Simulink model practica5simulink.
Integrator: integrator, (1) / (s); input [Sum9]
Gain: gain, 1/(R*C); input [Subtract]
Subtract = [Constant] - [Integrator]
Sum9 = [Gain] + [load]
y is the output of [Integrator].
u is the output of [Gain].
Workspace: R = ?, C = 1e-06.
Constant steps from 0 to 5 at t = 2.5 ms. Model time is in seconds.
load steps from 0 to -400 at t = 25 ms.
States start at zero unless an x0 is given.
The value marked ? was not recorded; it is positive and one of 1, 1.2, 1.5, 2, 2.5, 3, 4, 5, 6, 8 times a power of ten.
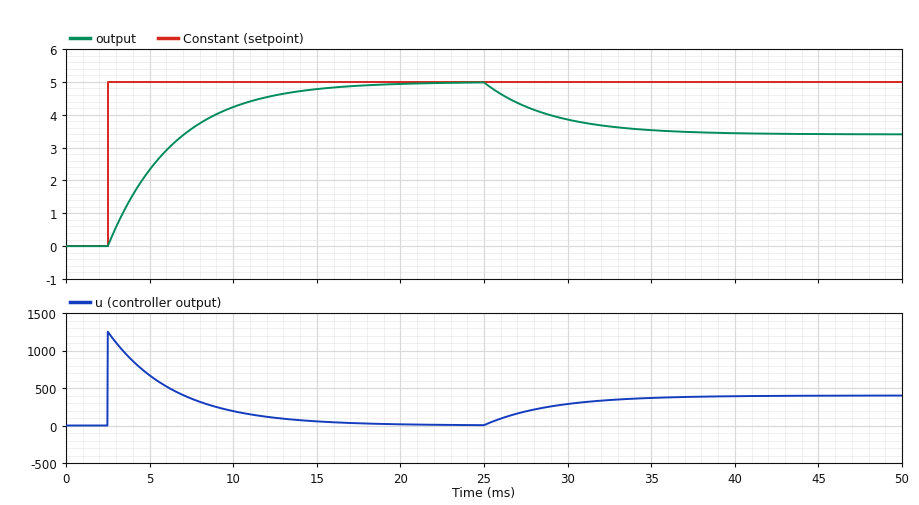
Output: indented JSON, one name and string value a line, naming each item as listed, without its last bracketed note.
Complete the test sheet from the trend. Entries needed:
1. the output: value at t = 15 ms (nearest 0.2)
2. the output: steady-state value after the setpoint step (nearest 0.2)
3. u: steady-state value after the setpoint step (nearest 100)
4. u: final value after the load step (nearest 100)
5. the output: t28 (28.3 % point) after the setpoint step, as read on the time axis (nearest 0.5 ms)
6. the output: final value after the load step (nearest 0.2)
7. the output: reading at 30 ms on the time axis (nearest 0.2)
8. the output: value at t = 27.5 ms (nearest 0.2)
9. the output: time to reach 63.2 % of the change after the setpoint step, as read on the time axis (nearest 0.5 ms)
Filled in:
{
  "the output: value at t = 15 ms": "4.8",
  "the output: steady-state value after the setpoint step": "5.0",
  "u: steady-state value after the setpoint step": "0",
  "u: final value after the load step": "400",
  "the output: t28 (28.3 % point) after the setpoint step, as read on the time axis": "4.0 ms",
  "the output: final value after the load step": "3.4",
  "the output: reading at 30 ms on the time axis": "3.8",
  "the output: value at t = 27.5 ms": "4.2",
  "the output: time to reach 63.2 % of the change after the setpoint step, as read on the time axis": "6.5 ms"
}
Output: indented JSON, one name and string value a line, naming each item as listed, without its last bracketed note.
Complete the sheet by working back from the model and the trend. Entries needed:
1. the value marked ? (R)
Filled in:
{
  "the value marked ?": "4000"
}
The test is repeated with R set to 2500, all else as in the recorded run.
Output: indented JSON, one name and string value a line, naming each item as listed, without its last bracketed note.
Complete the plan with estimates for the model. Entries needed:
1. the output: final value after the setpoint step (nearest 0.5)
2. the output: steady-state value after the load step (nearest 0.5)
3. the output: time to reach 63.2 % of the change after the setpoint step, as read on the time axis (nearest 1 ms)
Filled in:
{
  "the output: final value after the setpoint step": "5.0",
  "the output: steady-state value after the load step": "4.0",
  "the output: time to reach 63.2 % of the change after the setpoint step, as read on the time axis": "5 ms"
}
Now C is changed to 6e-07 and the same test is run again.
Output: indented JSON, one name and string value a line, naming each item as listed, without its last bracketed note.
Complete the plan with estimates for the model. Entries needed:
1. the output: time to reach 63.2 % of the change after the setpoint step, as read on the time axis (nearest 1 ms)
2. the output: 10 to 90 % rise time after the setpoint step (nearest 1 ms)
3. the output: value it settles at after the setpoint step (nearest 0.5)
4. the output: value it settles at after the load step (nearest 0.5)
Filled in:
{
  "the output: time to reach 63.2 % of the change after the setpoint step, as read on the time axis": "5 ms",
  "the output: 10 to 90 % rise time after the setpoint step": "5 ms",
  "the output: value it settles at after the setpoint step": "5.0",
  "the output: value it settles at after the load step": "4.0"
}
